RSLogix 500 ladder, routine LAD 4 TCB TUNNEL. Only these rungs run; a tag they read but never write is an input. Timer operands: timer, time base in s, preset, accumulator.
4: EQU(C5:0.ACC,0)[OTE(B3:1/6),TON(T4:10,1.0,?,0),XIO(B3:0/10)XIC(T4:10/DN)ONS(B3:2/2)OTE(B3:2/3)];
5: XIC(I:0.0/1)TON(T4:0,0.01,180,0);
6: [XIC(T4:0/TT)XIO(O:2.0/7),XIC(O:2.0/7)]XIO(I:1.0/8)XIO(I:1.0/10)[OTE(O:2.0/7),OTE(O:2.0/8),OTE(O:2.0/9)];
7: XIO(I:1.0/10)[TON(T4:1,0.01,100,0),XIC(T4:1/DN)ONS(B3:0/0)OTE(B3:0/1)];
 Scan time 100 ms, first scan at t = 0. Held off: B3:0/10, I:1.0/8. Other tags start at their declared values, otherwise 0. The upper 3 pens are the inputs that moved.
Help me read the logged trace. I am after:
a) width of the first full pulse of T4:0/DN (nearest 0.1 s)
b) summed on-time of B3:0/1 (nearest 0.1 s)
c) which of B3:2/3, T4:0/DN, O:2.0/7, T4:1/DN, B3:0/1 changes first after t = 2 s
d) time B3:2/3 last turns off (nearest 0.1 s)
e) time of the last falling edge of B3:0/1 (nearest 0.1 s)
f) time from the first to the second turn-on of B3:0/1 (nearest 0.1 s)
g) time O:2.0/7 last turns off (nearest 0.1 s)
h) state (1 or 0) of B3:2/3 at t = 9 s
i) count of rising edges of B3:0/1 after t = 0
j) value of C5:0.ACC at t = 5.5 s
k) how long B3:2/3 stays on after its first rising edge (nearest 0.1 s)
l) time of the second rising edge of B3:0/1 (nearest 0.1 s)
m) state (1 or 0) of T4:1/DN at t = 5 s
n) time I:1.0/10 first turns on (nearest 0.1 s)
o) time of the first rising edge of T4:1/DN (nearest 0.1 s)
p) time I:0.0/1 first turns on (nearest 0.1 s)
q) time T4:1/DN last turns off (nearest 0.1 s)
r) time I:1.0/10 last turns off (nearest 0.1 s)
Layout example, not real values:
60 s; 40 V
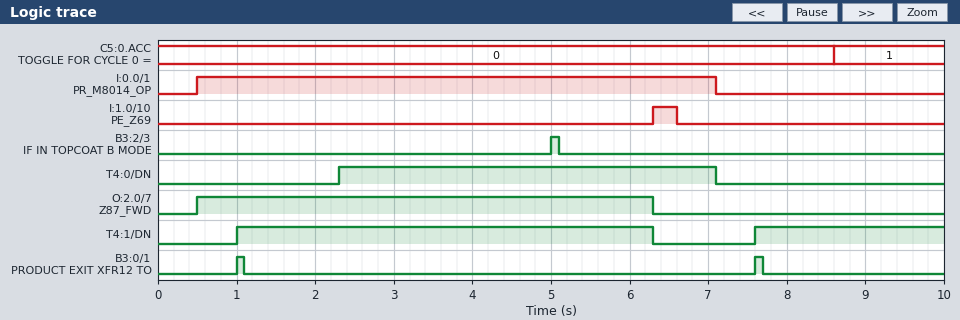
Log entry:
4.8 s; 0.2 s; T4:0/DN; 5.1 s; 7.7 s; 6.6 s; 6.3 s; 0; 2; 0; 0.1 s; 7.6 s; 1; 6.3 s; 1.0 s; 0.5 s; 6.3 s; 6.6 s
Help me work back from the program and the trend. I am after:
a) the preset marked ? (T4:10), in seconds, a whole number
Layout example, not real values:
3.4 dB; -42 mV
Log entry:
5 s
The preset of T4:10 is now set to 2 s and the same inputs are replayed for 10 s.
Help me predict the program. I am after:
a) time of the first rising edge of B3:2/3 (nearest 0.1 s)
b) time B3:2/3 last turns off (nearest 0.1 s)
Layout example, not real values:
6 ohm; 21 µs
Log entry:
2.0 s; 2.1 s
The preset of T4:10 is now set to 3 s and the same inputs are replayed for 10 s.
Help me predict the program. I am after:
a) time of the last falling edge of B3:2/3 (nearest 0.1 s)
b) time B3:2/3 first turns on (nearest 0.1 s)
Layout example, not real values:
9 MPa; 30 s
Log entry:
3.1 s; 3.0 s
